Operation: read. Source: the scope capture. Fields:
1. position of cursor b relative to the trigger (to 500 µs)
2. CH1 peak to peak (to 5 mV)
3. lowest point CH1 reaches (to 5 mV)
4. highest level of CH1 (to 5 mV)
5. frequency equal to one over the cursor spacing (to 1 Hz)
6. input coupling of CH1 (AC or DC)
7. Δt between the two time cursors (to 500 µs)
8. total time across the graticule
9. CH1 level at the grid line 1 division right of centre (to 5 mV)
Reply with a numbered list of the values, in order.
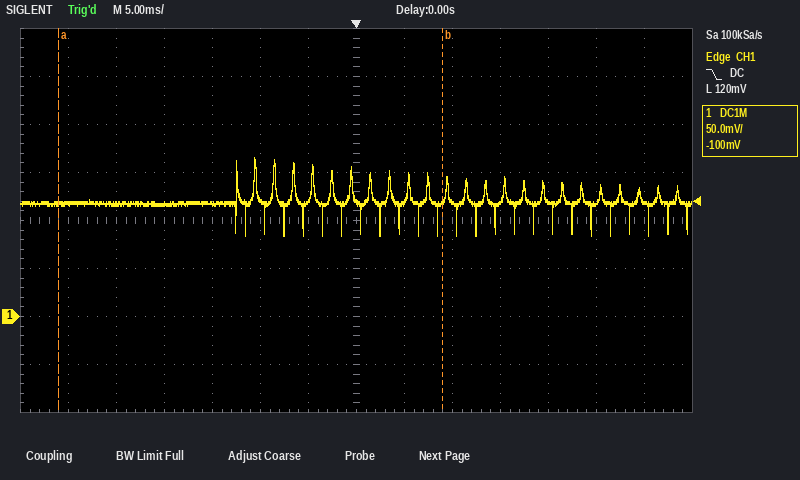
1. +9.0 ms
2. 80 mV
3. 85 mV
4. 165 mV
5. 25 Hz
6. DC
7. 40.0 ms
8. 70 ms
9. 120 mV
